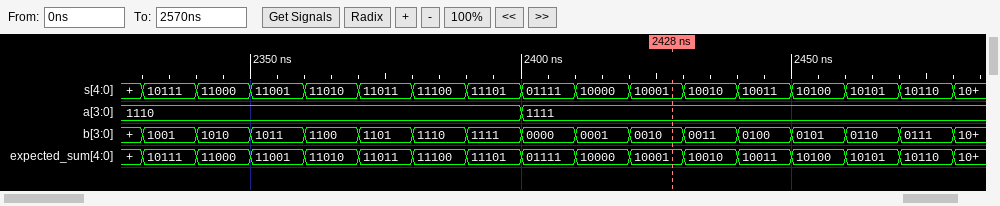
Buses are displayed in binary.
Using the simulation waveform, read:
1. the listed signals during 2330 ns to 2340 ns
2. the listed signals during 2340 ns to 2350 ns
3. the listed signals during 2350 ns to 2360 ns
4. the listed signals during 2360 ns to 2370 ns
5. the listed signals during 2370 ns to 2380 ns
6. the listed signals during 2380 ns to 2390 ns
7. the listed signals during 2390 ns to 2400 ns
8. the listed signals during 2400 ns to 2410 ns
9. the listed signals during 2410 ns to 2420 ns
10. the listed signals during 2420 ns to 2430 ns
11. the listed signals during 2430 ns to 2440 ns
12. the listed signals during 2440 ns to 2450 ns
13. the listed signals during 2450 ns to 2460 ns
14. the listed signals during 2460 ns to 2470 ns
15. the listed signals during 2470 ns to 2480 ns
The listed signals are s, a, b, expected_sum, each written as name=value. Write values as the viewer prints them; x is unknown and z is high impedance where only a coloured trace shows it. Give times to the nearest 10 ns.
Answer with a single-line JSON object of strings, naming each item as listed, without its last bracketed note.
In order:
{"the listed signals during 2330 ns to 2340 ns": "s=10111, a=1110, b=1001, expected_sum=10111", "the listed signals during 2340 ns to 2350 ns": "s=11000, a=1110, b=1010, expected_sum=11000", "the listed signals during 2350 ns to 2360 ns": "s=11001, a=1110, b=1011, expected_sum=11001", "the listed signals during 2360 ns to 2370 ns": "s=11010, a=1110, b=1100, expected_sum=11010", "the listed signals during 2370 ns to 2380 ns": "s=11011, a=1110, b=1101, expected_sum=11011", "the listed signals during 2380 ns to 2390 ns": "s=11100, a=1110, b=1110, expected_sum=11100", "the listed signals during 2390 ns to 2400 ns": "s=11101, a=1110, b=1111, expected_sum=11101", "the listed signals during 2400 ns to 2410 ns": "s=01111, a=1111, b=0000, expected_sum=01111", "the listed signals during 2410 ns to 2420 ns": "s=10000, a=1111, b=0001, expected_sum=10000", "the listed signals during 2420 ns to 2430 ns": "s=10001, a=1111, b=0010, expected_sum=10001", "the listed signals during 2430 ns to 2440 ns": "s=10010, a=1111, b=0011, expected_sum=10010", "the listed signals during 2440 ns to 2450 ns": "s=10011, a=1111, b=0100, expected_sum=10011", "the listed signals during 2450 ns to 2460 ns": "s=10100, a=1111, b=0101, expected_sum=10100", "the listed signals during 2460 ns to 2470 ns": "s=10101, a=1111, b=0110, expected_sum=10101", "the listed signals during 2470 ns to 2480 ns": "s=10110, a=1111, b=0111, expected_sum=10110"}
